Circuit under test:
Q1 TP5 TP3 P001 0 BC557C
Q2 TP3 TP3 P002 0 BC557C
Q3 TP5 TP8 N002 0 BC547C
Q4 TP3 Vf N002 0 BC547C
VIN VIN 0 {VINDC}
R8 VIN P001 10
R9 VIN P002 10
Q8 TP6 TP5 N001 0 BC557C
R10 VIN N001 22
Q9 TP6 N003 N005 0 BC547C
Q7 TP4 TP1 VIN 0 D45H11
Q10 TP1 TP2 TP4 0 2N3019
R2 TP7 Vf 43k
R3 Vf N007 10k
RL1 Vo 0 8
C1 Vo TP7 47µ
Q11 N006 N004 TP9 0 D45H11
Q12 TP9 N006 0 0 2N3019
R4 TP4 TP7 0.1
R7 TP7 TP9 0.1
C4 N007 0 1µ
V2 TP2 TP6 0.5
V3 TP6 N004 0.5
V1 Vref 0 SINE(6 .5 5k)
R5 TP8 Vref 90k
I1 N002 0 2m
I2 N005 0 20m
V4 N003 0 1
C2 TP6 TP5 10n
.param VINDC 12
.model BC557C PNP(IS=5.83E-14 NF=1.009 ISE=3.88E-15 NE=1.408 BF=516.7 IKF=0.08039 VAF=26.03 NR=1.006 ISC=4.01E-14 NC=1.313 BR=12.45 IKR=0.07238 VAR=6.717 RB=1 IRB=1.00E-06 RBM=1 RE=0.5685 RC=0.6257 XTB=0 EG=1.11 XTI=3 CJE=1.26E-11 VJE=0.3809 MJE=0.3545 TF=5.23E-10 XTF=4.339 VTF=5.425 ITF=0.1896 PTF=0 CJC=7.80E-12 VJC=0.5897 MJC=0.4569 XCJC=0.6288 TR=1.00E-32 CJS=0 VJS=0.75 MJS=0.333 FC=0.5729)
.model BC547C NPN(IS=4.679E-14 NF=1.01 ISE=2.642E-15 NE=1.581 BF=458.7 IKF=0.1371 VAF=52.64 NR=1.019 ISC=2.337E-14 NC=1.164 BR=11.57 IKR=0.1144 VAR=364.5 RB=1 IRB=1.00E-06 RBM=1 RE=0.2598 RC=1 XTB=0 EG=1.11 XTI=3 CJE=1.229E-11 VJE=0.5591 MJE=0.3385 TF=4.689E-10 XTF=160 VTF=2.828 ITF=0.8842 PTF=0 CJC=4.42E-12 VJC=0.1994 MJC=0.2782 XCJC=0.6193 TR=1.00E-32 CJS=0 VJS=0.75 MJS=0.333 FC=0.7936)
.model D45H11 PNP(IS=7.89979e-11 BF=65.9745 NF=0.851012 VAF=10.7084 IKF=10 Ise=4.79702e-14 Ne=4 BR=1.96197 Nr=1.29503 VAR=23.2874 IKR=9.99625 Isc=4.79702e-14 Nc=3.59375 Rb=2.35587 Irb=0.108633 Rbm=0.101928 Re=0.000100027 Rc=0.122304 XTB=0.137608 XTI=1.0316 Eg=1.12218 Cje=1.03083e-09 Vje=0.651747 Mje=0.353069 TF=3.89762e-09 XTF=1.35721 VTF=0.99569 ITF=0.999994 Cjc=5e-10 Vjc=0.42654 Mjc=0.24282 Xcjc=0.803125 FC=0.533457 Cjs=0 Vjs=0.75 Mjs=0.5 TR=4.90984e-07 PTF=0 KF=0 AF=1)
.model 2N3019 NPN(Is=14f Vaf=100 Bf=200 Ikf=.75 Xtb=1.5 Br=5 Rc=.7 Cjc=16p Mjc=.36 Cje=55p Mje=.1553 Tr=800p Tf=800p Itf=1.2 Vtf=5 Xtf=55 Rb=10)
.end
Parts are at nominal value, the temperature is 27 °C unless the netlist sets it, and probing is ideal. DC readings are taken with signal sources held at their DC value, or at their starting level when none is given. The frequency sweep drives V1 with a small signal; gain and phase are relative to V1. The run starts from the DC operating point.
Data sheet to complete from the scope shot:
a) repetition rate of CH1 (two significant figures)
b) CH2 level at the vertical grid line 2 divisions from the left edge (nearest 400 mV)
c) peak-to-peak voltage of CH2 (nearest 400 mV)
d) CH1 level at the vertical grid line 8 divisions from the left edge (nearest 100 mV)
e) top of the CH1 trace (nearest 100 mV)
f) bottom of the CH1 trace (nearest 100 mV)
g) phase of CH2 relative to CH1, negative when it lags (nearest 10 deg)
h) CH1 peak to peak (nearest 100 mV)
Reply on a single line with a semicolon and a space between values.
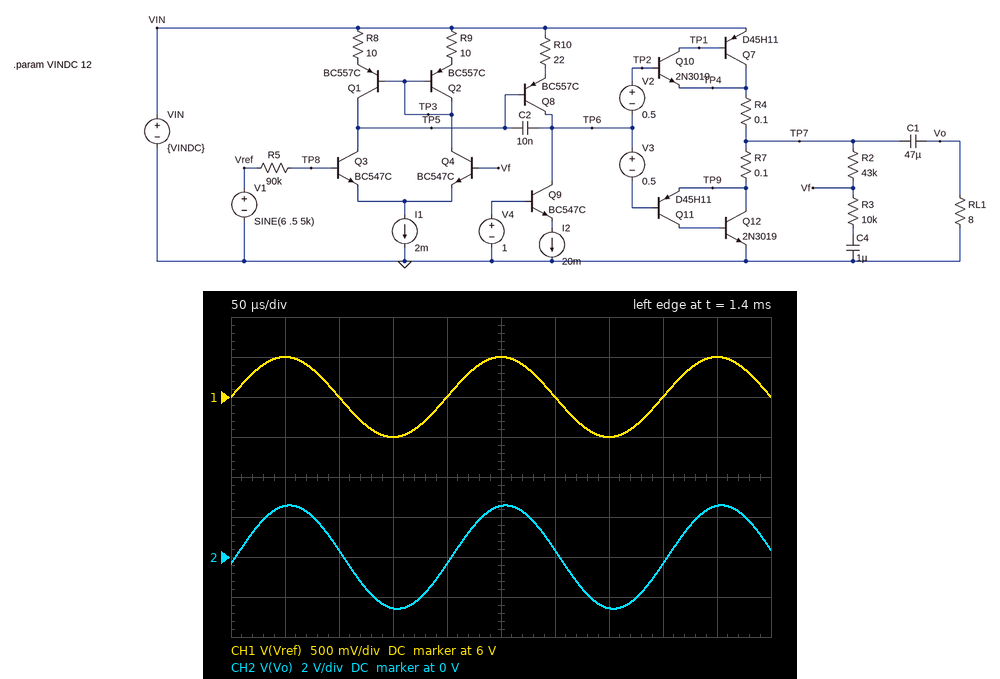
5.0 kHz; 400 mV; 5.2 V; 6.0 V; 6.5 V; 5.5 V; -10 deg; 1.0 V
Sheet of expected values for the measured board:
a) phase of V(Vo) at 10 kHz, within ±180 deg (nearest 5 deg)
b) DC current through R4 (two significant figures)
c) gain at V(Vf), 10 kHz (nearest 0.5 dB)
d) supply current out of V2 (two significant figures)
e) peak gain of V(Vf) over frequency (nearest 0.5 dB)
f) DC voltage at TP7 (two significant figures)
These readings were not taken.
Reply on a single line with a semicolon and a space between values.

-20 deg; 95 mA; -0.5 dB; 4.5 µA; 0 dB; 5.9 V
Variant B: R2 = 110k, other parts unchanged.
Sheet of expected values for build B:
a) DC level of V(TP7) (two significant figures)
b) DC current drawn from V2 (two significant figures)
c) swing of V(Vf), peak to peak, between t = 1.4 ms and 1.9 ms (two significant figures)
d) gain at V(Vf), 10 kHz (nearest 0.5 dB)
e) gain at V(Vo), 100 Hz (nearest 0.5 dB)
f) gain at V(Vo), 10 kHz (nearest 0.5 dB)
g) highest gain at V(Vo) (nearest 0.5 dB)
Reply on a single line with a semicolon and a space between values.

6.0 V; 4.6 µA; 870 mV; -3.0 dB; 8.5 dB; 19.0 dB; 21.0 dB
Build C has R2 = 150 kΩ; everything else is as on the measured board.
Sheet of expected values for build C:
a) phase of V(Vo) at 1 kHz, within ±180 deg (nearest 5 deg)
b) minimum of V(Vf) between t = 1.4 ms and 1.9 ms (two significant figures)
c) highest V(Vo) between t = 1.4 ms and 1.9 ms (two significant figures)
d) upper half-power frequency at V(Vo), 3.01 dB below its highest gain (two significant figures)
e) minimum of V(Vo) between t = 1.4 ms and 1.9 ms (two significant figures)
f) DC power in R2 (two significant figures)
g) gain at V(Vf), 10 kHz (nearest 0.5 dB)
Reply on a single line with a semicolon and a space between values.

15 deg; 5.5 V; 5.6 V; 8.7 kHz; -5.3 V; 560 nW; -4.0 dB
